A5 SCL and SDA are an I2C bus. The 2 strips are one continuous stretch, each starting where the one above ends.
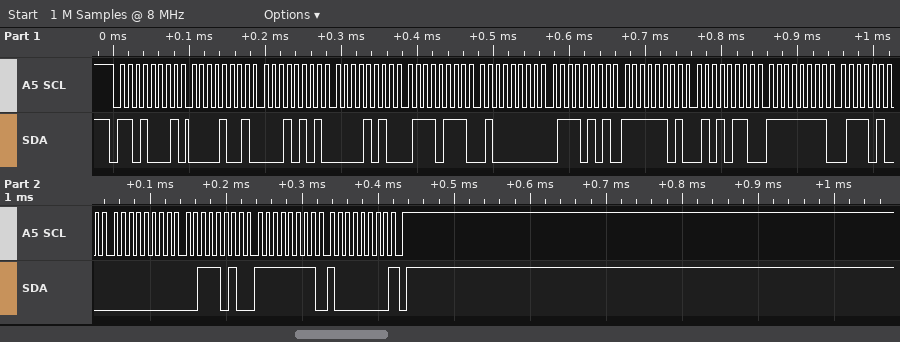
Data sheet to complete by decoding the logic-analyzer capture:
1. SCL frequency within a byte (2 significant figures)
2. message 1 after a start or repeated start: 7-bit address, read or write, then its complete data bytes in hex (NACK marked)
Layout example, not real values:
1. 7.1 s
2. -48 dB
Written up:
1. 100 kHz
2. 0x68 read: 09 15 0A 77 40 75 FD 56 FF 74 00 3A FF 80 NACK
